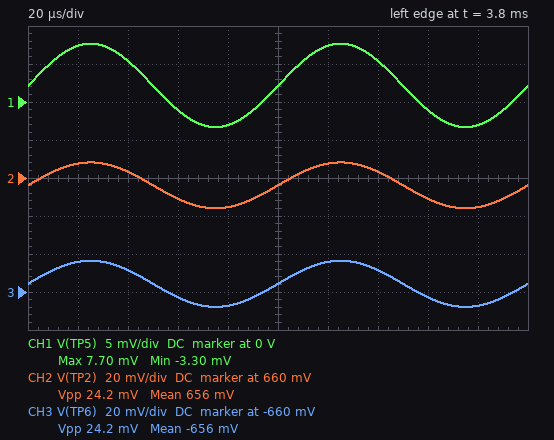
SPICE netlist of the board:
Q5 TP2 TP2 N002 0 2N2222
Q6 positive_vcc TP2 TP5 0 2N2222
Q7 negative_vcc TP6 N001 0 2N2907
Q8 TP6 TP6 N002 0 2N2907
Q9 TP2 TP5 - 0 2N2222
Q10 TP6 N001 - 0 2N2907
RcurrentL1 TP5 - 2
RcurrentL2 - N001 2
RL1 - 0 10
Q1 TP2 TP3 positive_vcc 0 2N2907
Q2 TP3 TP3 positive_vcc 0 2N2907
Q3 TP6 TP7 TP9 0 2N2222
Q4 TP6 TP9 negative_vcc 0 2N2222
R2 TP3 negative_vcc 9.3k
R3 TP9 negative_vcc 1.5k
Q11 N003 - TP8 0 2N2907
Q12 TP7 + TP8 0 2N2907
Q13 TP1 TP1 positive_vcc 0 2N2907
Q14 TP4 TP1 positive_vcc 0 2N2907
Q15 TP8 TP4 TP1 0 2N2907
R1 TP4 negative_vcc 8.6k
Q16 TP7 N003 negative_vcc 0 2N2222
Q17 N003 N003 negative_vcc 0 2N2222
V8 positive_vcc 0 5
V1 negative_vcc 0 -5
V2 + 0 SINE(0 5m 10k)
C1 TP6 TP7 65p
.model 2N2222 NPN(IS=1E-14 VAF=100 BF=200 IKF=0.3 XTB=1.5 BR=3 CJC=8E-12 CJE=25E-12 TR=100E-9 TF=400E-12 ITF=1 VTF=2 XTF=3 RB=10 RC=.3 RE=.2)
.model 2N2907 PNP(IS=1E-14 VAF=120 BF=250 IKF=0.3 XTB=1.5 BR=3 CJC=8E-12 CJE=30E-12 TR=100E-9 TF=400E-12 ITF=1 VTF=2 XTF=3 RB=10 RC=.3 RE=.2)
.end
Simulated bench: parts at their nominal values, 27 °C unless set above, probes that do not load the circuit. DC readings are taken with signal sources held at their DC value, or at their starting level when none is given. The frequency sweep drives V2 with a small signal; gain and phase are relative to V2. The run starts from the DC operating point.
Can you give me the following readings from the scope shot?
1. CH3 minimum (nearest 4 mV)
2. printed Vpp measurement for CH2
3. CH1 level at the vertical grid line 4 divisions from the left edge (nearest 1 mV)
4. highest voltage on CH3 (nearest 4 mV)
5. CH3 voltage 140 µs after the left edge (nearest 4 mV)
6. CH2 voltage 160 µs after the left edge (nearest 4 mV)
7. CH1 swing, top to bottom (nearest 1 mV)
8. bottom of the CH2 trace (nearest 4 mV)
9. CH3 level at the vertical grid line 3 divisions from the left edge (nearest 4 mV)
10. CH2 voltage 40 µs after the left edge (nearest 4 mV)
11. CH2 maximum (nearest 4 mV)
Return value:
-668 mV
24.2 mV
-3 mV
-644 mV
-648 mV
648 mV
11 mV
644 mV
-664 mV
664 mV
668 mV
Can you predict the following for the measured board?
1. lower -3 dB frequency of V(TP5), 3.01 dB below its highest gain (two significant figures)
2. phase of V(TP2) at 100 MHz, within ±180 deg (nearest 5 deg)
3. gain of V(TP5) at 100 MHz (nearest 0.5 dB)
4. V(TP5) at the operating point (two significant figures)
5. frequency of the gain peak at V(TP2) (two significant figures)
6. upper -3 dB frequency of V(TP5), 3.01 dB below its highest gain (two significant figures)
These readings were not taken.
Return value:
13 MHz
70 deg
-15.5 dB
2.1 mV
16 MHz
19 MHz
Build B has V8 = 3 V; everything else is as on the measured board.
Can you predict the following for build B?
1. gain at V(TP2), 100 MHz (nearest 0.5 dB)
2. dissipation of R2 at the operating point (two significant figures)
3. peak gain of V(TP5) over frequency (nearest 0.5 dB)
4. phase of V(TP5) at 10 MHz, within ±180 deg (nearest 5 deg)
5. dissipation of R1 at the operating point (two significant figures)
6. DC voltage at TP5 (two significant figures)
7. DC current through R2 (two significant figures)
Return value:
-16.5 dB
5.8 mW
8.5 dB
-90 deg
5.2 mW
1.7 mV
790 µA
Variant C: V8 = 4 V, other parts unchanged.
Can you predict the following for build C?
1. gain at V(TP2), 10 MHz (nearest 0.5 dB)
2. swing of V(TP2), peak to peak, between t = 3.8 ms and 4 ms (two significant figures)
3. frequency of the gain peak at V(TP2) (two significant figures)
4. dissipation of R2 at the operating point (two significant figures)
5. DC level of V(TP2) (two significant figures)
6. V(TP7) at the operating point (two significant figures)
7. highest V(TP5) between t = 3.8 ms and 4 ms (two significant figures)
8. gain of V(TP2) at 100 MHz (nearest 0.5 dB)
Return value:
13.5 dB
26 mV
13 MHz
7.5 mW
650 mV
-3.7 V
7.5 mV
-15.5 dB
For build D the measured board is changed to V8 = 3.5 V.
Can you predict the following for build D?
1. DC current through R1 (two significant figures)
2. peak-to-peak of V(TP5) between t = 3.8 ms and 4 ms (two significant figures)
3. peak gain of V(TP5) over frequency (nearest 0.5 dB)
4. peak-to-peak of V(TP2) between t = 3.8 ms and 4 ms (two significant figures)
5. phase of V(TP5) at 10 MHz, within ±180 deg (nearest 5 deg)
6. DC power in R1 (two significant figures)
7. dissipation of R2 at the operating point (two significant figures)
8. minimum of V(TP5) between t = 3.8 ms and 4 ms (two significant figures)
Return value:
840 µA
11 mV
9.0 dB
27 mV
-65 deg
6.0 mW
6.6 mW
-3.6 mV
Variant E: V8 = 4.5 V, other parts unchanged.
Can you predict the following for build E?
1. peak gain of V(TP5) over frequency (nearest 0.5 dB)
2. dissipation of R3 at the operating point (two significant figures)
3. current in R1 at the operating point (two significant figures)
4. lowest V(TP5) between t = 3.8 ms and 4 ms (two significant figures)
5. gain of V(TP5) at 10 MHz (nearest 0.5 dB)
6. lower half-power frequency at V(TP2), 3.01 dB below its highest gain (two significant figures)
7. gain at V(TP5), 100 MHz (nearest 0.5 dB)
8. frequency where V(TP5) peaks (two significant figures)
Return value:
10.5 dB
270 µW
950 µA
-3.4 mV
5.0 dB
12 MHz
-16.0 dB
15 MHz
